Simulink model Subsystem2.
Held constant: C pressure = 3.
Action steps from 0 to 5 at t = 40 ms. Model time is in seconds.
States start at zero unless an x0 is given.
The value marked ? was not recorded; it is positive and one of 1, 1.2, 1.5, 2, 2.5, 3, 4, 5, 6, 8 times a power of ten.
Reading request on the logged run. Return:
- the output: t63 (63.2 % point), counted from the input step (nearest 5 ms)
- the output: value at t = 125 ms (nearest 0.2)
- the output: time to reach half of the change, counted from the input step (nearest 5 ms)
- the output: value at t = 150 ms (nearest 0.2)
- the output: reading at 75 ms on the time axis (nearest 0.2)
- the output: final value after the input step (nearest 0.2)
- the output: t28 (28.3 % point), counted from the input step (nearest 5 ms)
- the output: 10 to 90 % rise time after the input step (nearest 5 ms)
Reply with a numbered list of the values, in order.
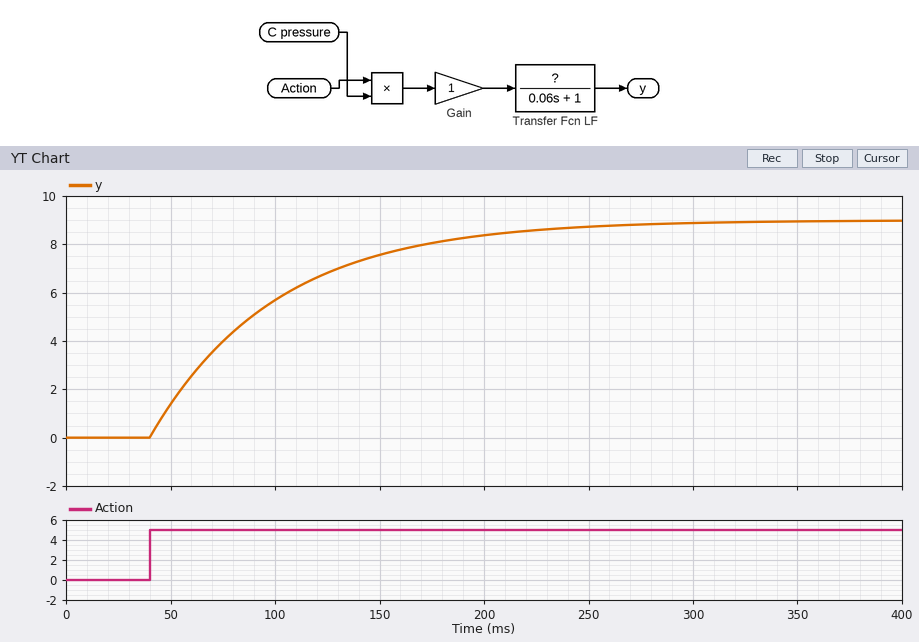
1. 60 ms
2. 6.8
3. 40 ms
4. 7.6
5. 4.0
6. 9.0
7. 20 ms
8. 130 ms
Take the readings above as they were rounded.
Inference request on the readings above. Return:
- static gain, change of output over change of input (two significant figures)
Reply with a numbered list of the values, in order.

1. 1.8
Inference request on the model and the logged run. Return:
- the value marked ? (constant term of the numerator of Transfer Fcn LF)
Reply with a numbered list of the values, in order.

1. 0.6
